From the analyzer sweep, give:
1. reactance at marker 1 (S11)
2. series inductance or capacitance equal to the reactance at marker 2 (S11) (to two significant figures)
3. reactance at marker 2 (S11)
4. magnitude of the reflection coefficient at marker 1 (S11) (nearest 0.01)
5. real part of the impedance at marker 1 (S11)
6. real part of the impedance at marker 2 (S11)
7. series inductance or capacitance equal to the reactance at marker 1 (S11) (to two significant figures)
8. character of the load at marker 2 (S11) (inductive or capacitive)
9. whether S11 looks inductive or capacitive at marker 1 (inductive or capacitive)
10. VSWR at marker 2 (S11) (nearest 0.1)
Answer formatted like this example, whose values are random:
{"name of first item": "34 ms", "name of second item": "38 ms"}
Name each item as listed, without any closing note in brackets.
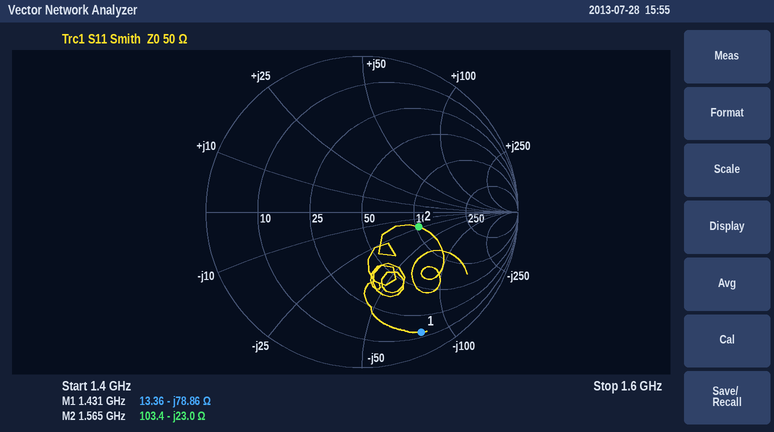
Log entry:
{"reactance at marker 1": "-78.86 Ω", "series inductance or capacitance equal to the reactance at marker 2 (S11)": "4.4 pF", "reactance at marker 2": "-23.0 Ω", "magnitude of the reflection coefficient at marker 1 (S11)": "0.86", "real part of the impedance at marker 1": "13.36 Ω", "real part of the impedance at marker 2": "103.4 Ω", "series inductance or capacitance equal to the reactance at marker 1 (S11)": "1.4 pF", "character of the load at marker 2 (S11)": "capacitive", "whether S11 looks inductive or capacitive at marker 1": "capacitive", "VSWR at marker 2 (S11)": "2.2"}
